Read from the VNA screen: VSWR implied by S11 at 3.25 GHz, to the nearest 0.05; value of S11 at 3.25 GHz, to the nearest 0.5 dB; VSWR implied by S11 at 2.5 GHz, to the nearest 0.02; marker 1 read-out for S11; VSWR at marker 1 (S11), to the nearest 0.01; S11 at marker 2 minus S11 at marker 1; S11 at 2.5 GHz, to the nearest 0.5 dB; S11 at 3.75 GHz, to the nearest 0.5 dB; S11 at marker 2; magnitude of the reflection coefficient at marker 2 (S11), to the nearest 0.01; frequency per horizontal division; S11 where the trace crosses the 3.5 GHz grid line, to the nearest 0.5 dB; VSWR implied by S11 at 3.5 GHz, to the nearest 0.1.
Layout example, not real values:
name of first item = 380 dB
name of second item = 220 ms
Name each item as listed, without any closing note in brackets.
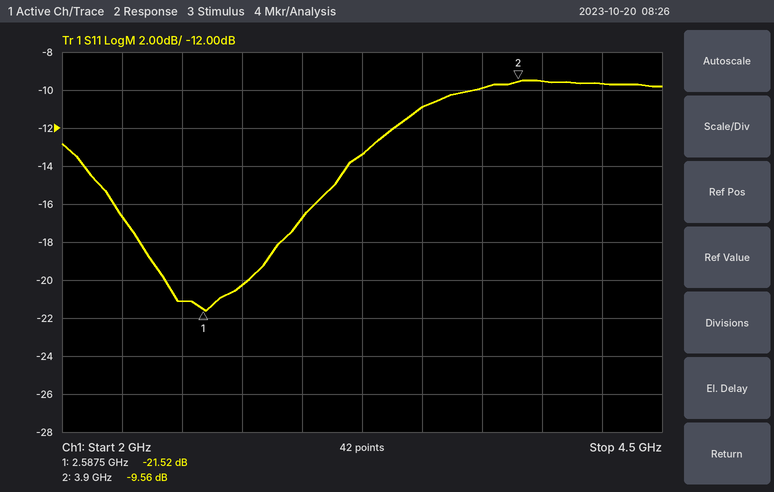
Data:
VSWR implied by S11 at 3.25 GHz, to the nearest 0.05 = 1.55
value of S11 at 3.25 GHz, to the nearest 0.5 dB = -13.5 dB
VSWR implied by S11 at 2.5 GHz, to the nearest 0.02 = 1.20
marker 1 read-out for S11 = -21.52 dB
VSWR at marker 1 (S11), to the nearest 0.01 = 1.18
S11 at marker 2 minus S11 at marker 1 = 11.96 dB
S11 at 2.5 GHz, to the nearest 0.5 dB = -21.0 dB
S11 at 3.75 GHz, to the nearest 0.5 dB = -10.0 dB
S11 at marker 2 = -9.56 dB
magnitude of the reflection coefficient at marker 2 (S11), to the nearest 0.01 = 0.33
frequency per horizontal division = 250 MHz
S11 where the trace crosses the 3.5 GHz grid line, to the nearest 0.5 dB = -11.0 dB
VSWR implied by S11 at 3.5 GHz, to the nearest 0.1 = 1.8
